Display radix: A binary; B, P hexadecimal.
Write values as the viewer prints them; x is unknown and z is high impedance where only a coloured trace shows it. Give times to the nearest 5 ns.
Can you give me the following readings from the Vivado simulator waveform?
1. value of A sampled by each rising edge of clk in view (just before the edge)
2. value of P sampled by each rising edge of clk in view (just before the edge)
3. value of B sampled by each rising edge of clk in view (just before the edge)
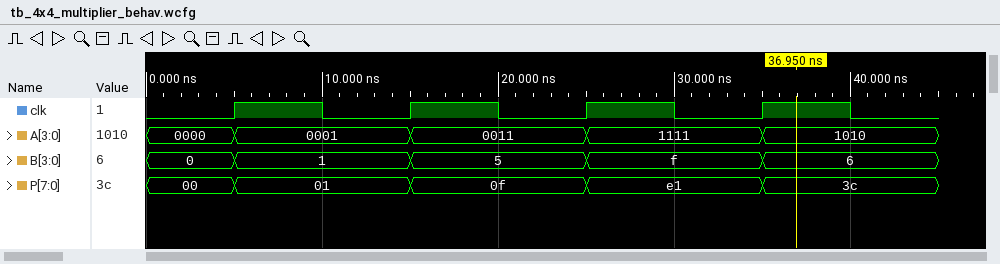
0000, 0001, 0011, 1111
00, 01, 0f, e1
0, 1, 5, f
